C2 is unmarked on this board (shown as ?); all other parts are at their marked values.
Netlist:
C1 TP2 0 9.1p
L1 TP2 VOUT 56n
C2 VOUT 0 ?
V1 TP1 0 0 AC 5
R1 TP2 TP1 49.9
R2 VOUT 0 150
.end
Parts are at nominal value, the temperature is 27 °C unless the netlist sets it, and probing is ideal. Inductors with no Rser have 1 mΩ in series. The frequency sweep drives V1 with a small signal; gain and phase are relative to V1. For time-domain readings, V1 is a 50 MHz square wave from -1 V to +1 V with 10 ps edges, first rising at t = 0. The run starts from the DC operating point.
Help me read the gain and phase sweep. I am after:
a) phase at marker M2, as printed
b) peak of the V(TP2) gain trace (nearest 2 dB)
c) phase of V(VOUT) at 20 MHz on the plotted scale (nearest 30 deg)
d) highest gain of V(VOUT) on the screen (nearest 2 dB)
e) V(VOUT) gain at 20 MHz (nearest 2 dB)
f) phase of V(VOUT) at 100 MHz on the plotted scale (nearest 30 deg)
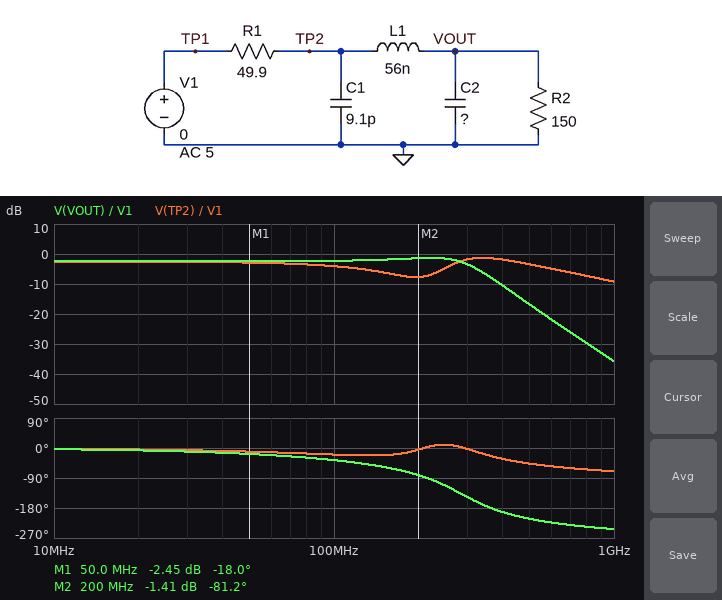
-81.2 deg
-2 dB
0 deg
-2 dB
-2 dB
-30 deg
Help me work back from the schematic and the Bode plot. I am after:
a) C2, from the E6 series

10 pF
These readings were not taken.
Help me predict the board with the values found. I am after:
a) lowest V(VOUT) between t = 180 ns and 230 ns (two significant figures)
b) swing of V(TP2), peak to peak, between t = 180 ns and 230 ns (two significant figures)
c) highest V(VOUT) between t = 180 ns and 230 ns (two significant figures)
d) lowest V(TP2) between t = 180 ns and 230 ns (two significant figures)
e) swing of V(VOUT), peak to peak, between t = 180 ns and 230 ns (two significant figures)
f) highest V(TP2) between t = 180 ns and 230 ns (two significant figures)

-1.0 V
1.7 V
1.0 V
-840 mV
2.0 V
840 mV
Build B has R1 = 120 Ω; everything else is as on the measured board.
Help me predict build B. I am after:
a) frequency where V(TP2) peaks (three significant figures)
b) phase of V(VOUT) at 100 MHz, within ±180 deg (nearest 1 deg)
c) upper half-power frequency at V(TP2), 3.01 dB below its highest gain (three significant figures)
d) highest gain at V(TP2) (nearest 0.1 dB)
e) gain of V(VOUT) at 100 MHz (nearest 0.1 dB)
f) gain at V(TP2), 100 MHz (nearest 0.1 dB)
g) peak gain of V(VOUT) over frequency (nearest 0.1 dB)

322 MHz
-47 deg
414 MHz
-3.3 dB
-6.4 dB
-8.2 dB
-5.1 dB
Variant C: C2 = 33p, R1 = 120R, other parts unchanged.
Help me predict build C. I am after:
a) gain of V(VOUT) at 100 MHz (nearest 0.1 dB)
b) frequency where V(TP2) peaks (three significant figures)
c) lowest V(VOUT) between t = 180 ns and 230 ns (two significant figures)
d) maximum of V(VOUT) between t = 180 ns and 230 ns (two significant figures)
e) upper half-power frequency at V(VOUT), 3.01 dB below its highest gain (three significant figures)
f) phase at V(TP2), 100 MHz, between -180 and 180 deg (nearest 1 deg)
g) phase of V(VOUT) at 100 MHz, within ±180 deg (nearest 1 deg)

-9.7 dB
255 MHz
-520 mV
520 mV
66.6 MHz
-32 deg
-73 deg
